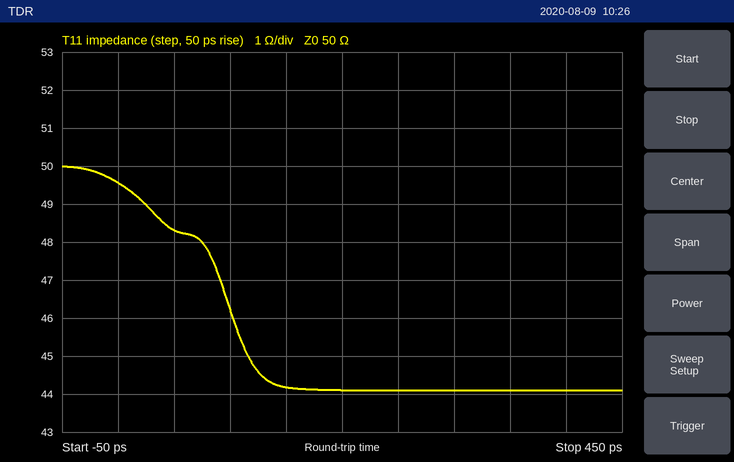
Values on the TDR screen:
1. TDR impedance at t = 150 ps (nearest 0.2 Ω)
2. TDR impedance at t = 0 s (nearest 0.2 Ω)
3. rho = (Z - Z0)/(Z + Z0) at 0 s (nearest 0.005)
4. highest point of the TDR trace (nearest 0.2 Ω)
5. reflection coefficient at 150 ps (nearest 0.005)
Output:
44.2 Ω
49.6 Ω
-0.005
50.0 Ω
-0.060
